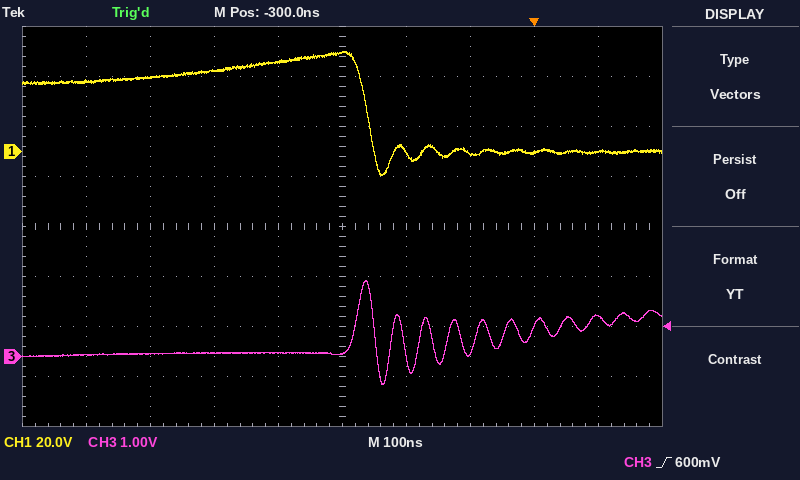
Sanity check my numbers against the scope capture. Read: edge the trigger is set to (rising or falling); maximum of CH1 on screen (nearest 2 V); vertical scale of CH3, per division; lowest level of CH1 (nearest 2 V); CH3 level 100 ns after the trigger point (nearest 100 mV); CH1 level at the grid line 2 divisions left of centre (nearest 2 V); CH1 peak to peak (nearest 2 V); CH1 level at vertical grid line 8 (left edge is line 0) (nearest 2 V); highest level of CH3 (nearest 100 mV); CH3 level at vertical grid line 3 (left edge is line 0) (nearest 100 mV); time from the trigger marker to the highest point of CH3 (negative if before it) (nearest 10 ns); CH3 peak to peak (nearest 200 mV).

rising
40 V
1 V
-10 V
800 mV
32 V
50 V
0 V
1.5 V
100 mV
-260 ns
2.0 V
